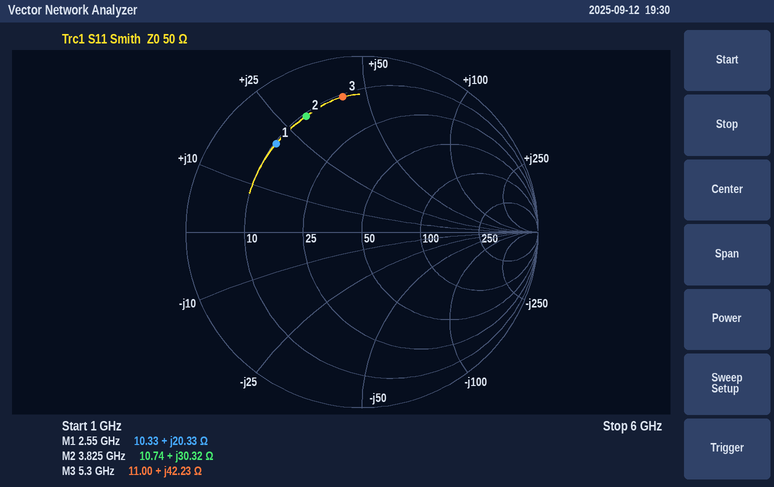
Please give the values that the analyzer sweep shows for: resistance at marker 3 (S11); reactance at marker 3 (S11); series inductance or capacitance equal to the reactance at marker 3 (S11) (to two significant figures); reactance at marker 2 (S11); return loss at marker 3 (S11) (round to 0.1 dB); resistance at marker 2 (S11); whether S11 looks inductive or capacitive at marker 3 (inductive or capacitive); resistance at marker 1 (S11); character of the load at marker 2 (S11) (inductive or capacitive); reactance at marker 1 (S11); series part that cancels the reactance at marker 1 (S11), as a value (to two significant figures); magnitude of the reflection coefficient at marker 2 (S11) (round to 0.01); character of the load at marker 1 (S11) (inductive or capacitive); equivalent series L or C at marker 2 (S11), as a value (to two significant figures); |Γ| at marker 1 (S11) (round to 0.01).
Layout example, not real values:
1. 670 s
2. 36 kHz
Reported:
1. 11.00 Ω
2. +42.23 Ω
3. 1.3 nH
4. +30.32 Ω
5. 2.2 dB
6. 10.74 Ω
7. inductive
8. 10.33 Ω
9. inductive
10. +20.33 Ω
11. 3.1 pF
12. 0.73
13. inductive
14. 1.3 nH
15. 0.70
